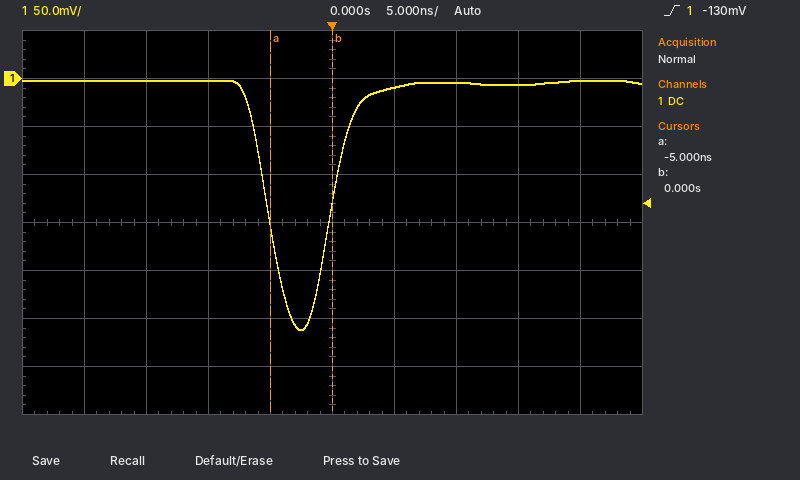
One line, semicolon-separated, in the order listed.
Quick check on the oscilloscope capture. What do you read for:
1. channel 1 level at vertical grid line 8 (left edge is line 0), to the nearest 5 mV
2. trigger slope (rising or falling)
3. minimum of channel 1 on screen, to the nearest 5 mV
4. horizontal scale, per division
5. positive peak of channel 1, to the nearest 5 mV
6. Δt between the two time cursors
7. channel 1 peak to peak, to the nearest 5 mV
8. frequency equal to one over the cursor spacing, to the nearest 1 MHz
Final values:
-5 mV; rising; -260 mV; 5 ns; 0 mV; 5.0 ns; 260 mV; 200 MHz
